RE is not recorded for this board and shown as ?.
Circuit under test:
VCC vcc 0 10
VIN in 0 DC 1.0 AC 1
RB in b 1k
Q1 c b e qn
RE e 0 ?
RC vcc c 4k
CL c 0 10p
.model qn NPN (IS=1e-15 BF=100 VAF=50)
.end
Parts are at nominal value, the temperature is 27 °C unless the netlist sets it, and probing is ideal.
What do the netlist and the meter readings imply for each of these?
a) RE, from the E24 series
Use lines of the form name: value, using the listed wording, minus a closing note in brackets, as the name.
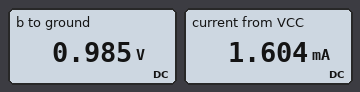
RE, from the E24 series: 160 Ω
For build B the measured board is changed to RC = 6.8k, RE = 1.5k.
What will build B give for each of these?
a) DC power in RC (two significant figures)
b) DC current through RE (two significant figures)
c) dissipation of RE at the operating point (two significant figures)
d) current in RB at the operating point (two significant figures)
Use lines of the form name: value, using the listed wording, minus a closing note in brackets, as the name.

DC power in RC: 320 µW
DC current through RE: 220 µA
dissipation of RE at the operating point: 71 µW
current in RB at the operating point: 1.9 µA
